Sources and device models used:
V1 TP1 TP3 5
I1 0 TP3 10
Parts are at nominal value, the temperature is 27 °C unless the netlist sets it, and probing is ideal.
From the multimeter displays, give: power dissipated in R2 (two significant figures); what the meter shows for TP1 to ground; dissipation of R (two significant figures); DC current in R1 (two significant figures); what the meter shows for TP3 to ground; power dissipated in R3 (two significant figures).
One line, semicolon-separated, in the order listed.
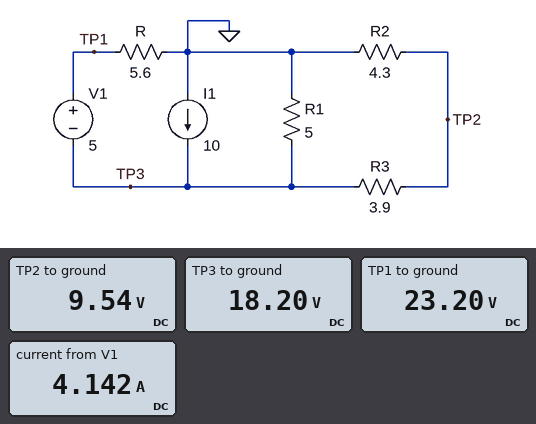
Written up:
21 W; 23.20 V; 96 W; 3.6 A; 18.20 V; 19 W
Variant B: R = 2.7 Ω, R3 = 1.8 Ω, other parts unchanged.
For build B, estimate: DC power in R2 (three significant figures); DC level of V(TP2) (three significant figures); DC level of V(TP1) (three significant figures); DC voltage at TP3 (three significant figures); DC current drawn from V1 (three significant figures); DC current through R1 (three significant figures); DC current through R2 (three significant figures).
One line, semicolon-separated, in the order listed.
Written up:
14.2 W; 7.82 V; 16.1 V; 11.1 V; 5.96 A; 2.22 A; 1.82 A
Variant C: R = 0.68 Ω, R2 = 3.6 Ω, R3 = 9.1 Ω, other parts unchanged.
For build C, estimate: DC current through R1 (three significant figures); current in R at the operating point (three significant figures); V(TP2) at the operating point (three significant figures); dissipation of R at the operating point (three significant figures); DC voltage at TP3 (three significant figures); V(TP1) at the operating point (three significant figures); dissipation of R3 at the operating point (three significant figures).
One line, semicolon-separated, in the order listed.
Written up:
303 mA; 9.58 A; 429 mV; 62.4 W; 1.51 V; 6.51 V; 129 mW
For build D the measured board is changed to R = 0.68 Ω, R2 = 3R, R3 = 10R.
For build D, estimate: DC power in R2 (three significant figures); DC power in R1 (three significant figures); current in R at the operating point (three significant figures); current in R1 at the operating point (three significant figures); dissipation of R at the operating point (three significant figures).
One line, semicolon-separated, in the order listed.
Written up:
40.7 mW; 459 mW; 9.58 A; 303 mA; 62.4 W
